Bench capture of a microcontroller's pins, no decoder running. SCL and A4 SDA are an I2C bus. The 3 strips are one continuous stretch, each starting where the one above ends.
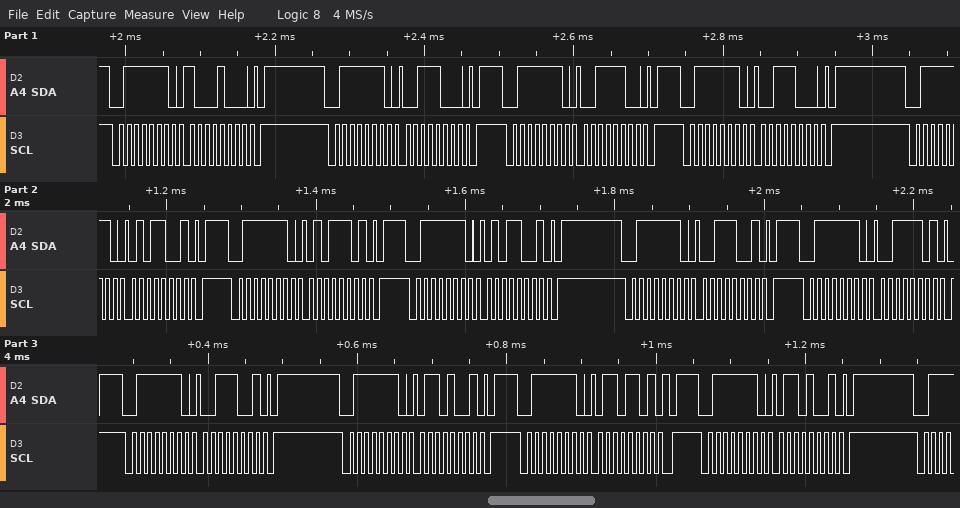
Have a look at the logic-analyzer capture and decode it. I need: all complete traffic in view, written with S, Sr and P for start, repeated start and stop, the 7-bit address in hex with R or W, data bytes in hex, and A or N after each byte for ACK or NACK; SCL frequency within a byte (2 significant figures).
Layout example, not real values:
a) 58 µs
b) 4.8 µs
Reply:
a) S 3FW A 88 A P S 3FW A 38 A P S 3FW A 3C A P S 3FW A 38 A P S 3FW A 59 A P S 3FW A 5D A P S 3FW A 59 A P S 3FW A 39 A P S 3FW A 3D A P S 3FW A 39 A P S 3FW A 69 A P S 3FW A 6D A P S 3FW A 69 A P
b) 100 kHz
